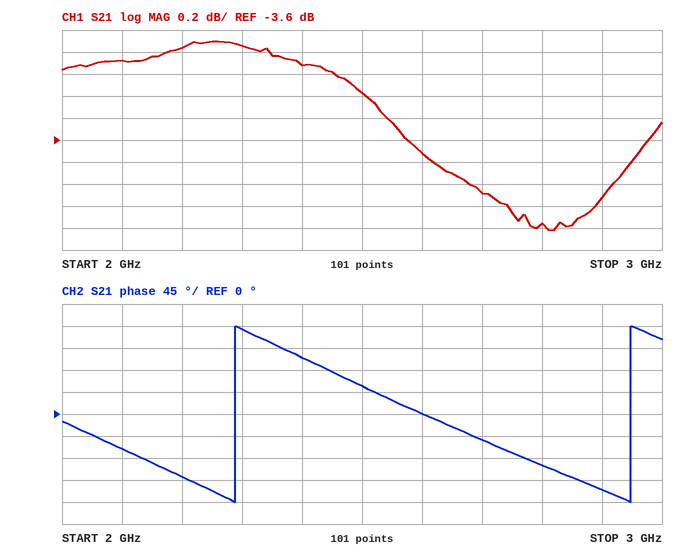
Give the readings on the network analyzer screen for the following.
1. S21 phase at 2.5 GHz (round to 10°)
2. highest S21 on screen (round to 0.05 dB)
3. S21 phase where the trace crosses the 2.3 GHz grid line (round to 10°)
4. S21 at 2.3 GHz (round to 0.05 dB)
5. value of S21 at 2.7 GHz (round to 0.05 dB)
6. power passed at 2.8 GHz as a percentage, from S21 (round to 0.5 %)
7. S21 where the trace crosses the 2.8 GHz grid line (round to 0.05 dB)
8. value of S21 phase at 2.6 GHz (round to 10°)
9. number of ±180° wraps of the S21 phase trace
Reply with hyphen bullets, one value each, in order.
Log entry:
- 60°
- -2.70 dB
- 170°
- -2.75 dB
- -4.10 dB
- 36.5 %
- -4.35 dB
- 0°
- 2
